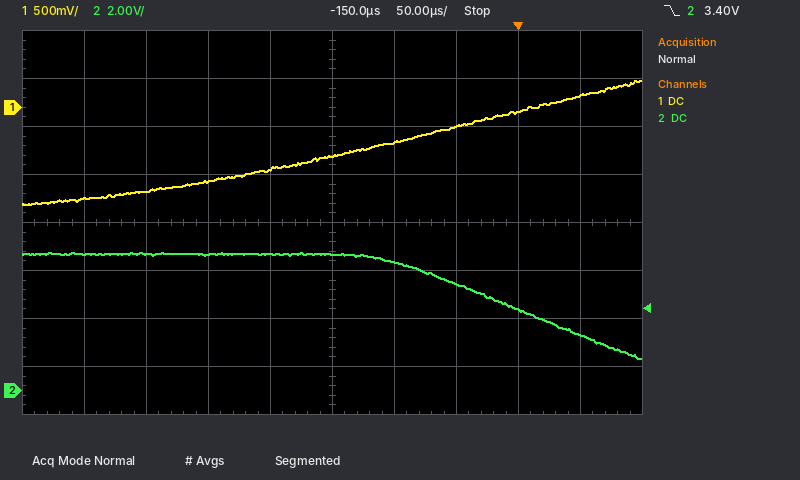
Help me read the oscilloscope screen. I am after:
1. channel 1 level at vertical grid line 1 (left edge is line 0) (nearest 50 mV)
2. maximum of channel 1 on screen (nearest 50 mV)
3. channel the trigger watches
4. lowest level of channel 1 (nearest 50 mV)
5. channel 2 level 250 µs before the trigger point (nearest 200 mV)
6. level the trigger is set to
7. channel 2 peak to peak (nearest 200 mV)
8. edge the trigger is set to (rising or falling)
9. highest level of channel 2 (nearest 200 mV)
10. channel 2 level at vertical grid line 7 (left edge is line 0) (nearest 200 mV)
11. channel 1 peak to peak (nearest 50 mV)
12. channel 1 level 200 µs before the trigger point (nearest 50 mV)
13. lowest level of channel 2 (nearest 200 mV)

-950 mV
300 mV
channel 2
-1.00 V
5.6 V
3.40 V
4.4 V
falling
5.8 V
4.4 V
1.30 V
-650 mV
1.4 V
